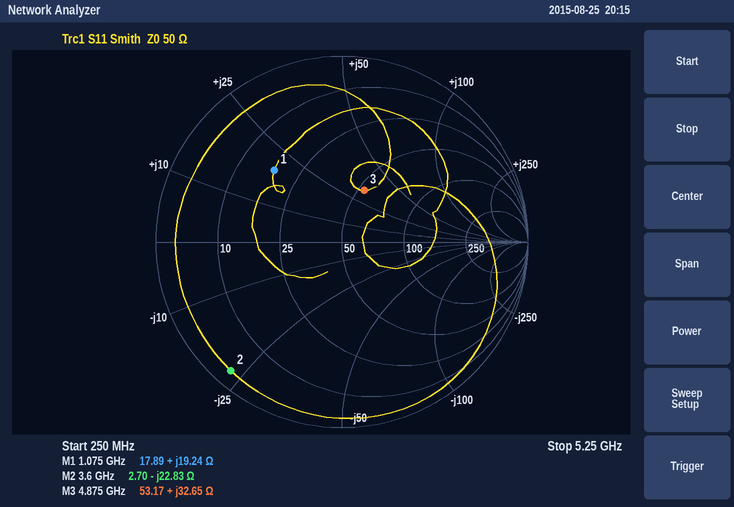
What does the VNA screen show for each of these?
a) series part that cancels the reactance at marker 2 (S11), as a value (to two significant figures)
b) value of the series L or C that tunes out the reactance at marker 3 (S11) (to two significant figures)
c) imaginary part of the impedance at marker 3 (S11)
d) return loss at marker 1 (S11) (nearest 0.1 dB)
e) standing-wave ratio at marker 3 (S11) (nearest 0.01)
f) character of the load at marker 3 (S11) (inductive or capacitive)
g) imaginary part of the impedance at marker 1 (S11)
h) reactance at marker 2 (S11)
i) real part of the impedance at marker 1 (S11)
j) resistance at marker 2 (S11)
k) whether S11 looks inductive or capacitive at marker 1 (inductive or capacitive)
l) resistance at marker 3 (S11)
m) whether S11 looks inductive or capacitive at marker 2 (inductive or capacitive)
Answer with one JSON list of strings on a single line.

["1.0 nH", "1.0 pF", "+32.65 Ω", "5.5 dB", "1.87", "inductive", "+19.24 Ω", "-22.83 Ω", "17.89 Ω", "2.70 Ω", "inductive", "53.17 Ω", "capacitive"]
